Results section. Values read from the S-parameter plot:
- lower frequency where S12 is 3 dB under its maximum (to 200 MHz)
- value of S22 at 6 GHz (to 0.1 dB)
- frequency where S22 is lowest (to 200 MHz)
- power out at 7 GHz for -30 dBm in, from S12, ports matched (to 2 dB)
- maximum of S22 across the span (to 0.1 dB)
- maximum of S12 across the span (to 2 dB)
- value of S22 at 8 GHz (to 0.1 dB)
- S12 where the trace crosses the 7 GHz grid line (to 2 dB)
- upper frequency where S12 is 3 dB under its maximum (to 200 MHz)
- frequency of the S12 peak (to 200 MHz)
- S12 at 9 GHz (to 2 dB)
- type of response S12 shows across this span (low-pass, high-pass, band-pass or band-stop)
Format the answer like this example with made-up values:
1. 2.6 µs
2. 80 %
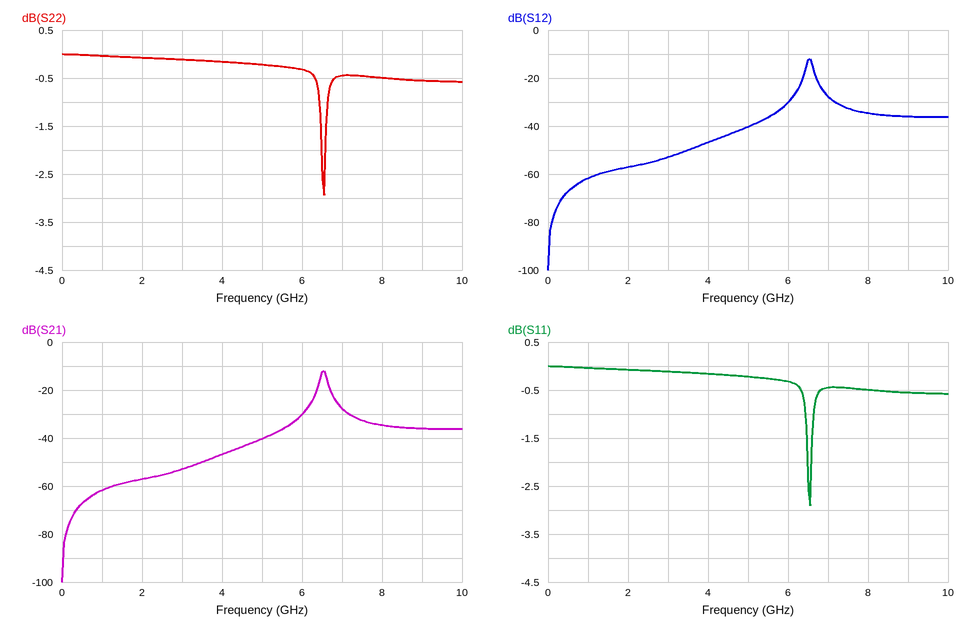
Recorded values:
1. 6.4 GHz
2. -0.3 dB
3. 6.6 GHz
4. -58 dBm
5. 0.0 dB
6. -12 dB
7. -0.5 dB
8. -28 dB
9. 6.6 GHz
10. 6.6 GHz
11. -36 dB
12. band-pass
